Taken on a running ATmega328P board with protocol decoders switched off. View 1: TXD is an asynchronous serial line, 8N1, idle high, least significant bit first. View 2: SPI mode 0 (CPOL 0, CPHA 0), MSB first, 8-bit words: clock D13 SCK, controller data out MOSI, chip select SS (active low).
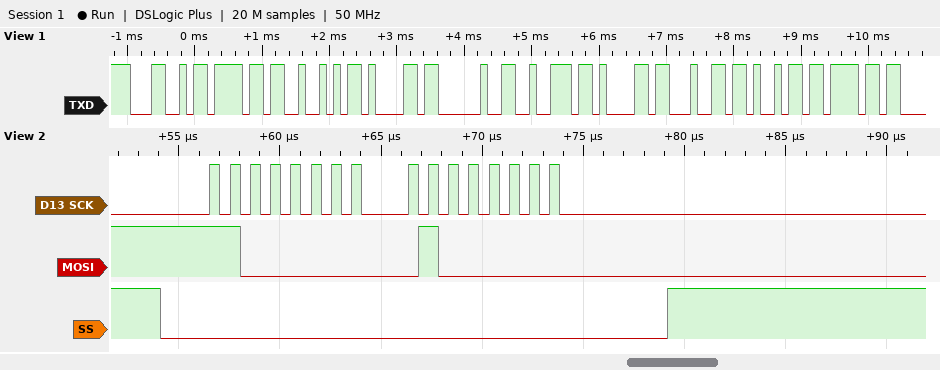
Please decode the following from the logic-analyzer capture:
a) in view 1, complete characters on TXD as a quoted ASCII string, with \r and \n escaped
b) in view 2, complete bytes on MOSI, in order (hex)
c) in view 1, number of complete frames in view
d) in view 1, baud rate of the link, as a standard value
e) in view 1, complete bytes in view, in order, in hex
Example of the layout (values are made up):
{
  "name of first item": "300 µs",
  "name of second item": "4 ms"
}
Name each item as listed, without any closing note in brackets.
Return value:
{
  "in view 1, complete characters on TXD as a quoted ASCII string, with \\r and \\n escaped": "\"LoRa radio\"",
  "in view 2, complete bytes on MOSI, in order": "C0 40",
  "in view 1, number of complete frames in view": "10",
  "in view 1, baud rate of the link, as a standard value": "9600 baud",
  "in view 1, complete bytes in view, in order, in hex": "0x4C 0x6F 0x52 0x61 0x20 0x72 0x61 0x64 0x69 0x6F"
}
